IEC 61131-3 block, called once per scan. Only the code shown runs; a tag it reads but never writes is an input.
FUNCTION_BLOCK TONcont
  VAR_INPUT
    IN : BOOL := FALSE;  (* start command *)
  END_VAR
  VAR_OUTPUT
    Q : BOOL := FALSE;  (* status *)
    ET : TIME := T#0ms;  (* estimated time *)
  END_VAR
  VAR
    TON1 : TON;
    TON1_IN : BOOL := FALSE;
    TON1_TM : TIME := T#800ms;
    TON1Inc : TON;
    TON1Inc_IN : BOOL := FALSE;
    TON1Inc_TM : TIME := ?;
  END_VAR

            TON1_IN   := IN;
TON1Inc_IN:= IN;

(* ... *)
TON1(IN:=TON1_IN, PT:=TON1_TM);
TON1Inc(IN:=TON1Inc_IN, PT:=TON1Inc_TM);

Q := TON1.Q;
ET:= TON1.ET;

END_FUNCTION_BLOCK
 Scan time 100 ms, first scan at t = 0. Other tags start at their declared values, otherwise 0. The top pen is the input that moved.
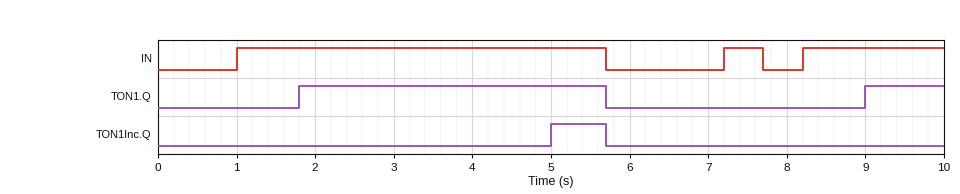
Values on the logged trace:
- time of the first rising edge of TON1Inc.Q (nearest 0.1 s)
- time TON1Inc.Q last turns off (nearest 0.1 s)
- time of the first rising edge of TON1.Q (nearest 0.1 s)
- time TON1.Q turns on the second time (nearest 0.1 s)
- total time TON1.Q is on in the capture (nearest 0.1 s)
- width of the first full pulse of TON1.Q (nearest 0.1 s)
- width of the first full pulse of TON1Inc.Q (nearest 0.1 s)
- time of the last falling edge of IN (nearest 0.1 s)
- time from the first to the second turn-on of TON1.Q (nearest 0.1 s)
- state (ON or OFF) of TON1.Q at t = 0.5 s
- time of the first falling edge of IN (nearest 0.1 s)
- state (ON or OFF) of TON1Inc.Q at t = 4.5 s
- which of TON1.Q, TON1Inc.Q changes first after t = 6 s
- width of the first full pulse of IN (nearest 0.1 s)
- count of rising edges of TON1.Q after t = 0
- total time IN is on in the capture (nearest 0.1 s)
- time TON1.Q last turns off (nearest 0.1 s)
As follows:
5.0 s
5.7 s
1.8 s
9.0 s
4.9 s
3.9 s
0.7 s
7.7 s
7.2 s
OFF
5.7 s
OFF
TON1.Q
4.7 s
2
7.0 s
5.7 s
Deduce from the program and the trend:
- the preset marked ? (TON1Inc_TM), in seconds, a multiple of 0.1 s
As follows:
4.0 s
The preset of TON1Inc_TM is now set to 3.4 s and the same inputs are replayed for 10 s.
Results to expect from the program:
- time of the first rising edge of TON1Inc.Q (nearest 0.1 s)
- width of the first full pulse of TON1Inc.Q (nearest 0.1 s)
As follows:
4.4 s
1.3 s
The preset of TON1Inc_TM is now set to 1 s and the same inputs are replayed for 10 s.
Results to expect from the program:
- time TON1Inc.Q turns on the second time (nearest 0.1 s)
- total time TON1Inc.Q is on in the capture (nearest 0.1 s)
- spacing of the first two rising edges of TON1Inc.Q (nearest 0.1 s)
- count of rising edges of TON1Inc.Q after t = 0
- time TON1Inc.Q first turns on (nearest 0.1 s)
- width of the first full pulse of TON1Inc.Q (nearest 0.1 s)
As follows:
9.2 s
4.5 s
7.2 s
2
2.0 s
3.7 s
